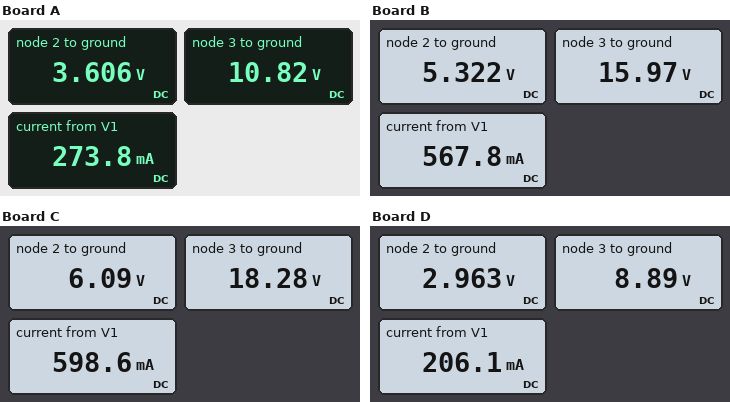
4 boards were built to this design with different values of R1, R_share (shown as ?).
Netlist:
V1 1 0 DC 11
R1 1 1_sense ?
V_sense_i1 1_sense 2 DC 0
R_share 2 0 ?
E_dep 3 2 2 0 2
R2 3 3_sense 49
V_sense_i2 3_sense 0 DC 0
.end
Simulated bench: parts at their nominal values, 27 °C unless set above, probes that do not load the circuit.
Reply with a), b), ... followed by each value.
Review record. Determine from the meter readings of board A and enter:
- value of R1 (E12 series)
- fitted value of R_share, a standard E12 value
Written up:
a) 27 Ω
b) 68 Ω
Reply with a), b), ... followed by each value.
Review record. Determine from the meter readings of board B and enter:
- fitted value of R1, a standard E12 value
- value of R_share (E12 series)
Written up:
a) 10 Ω
b) 22 Ω
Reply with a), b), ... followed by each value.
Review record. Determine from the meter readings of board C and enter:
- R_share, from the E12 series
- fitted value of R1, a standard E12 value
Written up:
a) 27 Ω
b) 8.2 Ω
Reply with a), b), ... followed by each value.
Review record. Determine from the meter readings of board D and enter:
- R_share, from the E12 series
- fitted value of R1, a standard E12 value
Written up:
a) 120 Ω
b) 39 Ω
